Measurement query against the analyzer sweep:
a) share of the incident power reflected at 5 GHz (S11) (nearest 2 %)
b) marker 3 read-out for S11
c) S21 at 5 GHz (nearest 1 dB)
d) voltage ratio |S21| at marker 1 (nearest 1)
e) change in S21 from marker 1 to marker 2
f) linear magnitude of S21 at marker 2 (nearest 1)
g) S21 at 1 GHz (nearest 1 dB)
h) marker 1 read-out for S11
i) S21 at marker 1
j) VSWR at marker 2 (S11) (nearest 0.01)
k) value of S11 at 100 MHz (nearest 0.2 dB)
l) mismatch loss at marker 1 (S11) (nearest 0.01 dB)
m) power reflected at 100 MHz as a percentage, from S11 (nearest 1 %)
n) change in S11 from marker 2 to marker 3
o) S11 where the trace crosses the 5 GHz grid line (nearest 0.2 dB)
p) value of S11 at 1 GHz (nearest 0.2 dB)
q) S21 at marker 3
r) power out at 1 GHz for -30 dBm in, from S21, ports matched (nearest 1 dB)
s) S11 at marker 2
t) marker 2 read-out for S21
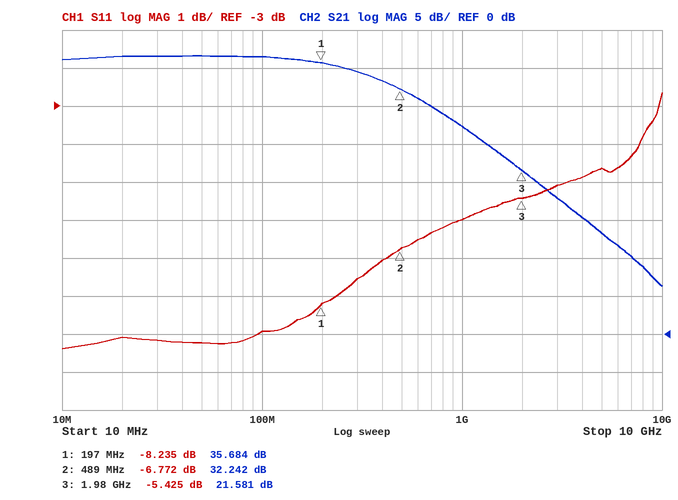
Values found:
34 %
-5.425 dB
13 dB
61
-3.442 dB
41
27 dB
-8.235 dB
35.684 dB
2.69
-9.0 dB
0.71 dB
13 %
1.347 dB
-4.6 dB
-6.0 dB
21.581 dB
-3 dBm
-6.772 dB
32.242 dB
